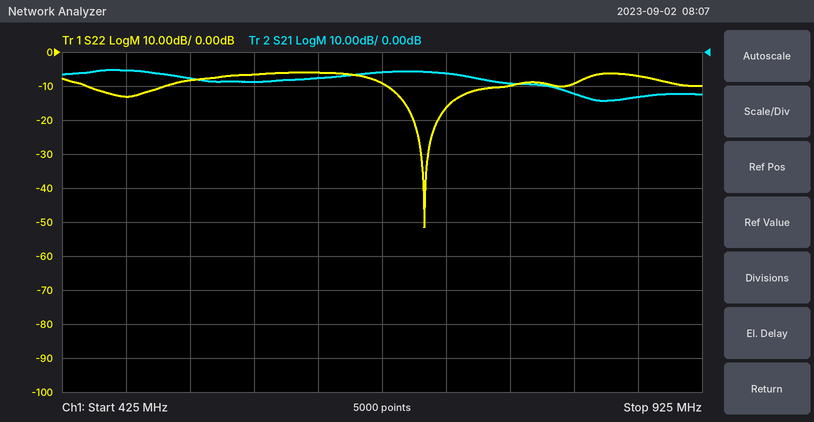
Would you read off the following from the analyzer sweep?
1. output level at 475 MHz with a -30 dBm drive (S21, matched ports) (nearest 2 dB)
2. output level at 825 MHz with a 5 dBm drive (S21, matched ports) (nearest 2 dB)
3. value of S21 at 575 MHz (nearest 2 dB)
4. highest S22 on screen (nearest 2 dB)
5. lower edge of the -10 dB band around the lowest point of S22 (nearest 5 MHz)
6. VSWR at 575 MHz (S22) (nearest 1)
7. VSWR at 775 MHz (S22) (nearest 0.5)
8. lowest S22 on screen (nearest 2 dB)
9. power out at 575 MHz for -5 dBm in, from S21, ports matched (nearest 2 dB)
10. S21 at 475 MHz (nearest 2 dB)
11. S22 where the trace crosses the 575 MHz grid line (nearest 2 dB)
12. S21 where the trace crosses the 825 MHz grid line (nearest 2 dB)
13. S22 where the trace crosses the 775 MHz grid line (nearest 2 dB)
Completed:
-36 dBm
-8 dBm
-8 dB
-6 dB
680 MHz
3
2.0
-52 dB
-14 dBm
-6 dB
-6 dB
-12 dB
-10 dB
